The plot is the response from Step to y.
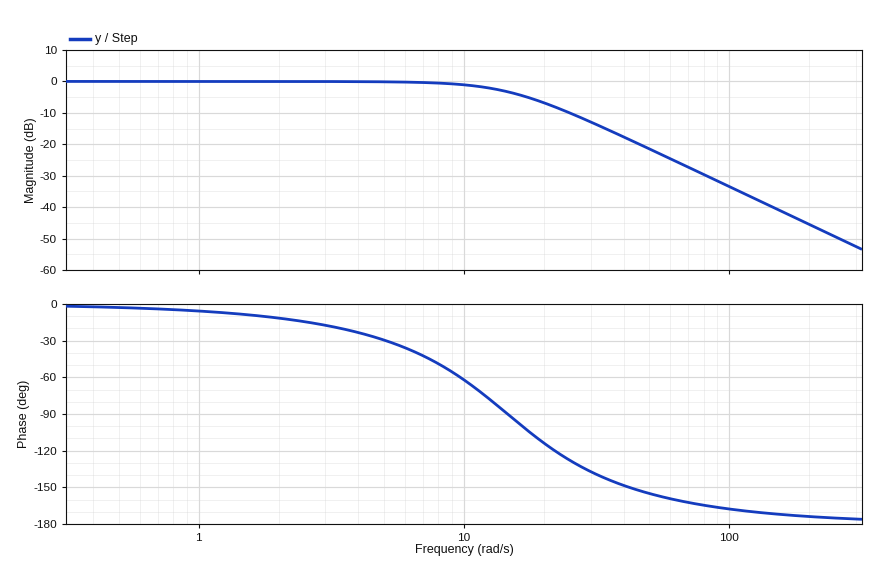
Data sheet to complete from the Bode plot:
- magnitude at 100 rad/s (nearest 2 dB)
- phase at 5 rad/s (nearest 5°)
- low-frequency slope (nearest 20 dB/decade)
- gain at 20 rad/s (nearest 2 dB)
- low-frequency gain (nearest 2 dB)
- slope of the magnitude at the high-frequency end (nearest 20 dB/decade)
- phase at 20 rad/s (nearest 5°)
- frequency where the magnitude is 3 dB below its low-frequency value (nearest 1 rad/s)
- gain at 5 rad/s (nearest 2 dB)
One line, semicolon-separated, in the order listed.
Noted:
-34 dB; -30°; 0 dB/decade; -6 dB; 0 dB; -40 dB/decade; -115°; 14 rad/s; 0 dB
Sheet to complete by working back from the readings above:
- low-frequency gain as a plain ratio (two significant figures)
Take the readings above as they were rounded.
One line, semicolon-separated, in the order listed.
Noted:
1.0
